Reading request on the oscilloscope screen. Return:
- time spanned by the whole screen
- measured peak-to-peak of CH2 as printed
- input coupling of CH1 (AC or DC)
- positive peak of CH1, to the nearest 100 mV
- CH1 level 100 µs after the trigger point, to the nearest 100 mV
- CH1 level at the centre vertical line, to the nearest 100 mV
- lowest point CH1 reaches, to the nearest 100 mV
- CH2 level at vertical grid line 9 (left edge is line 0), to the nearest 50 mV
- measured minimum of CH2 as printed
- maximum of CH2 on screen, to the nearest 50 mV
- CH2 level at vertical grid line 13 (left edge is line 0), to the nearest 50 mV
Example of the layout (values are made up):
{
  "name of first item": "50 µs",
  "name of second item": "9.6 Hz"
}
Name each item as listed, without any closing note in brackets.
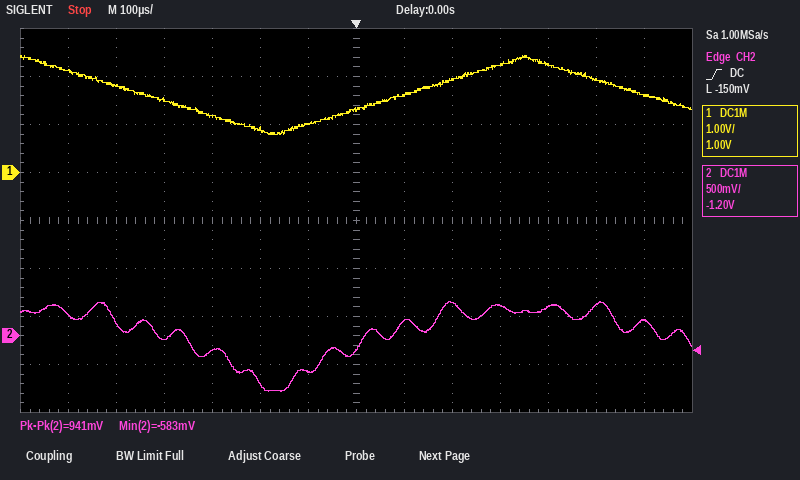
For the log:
{
  "time spanned by the whole screen": "1.4 ms",
  "measured peak-to-peak of CH2 as printed": "941 mV",
  "input coupling of CH1": "DC",
  "positive peak of CH1, to the nearest 100 mV": "2.4 V",
  "CH1 level 100 µs after the trigger point, to the nearest 100 mV": "1.6 V",
  "CH1 level at the centre vertical line, to the nearest 100 mV": "1.3 V",
  "lowest point CH1 reaches, to the nearest 100 mV": "800 mV",
  "CH2 level at vertical grid line 9 (left edge is line 0), to the nearest 50 mV": "350 mV",
  "measured minimum of CH2 as printed": "-583 mV",
  "maximum of CH2 on screen, to the nearest 50 mV": "350 mV",
  "CH2 level at vertical grid line 13 (left edge is line 0), to the nearest 50 mV": "150 mV"
}
